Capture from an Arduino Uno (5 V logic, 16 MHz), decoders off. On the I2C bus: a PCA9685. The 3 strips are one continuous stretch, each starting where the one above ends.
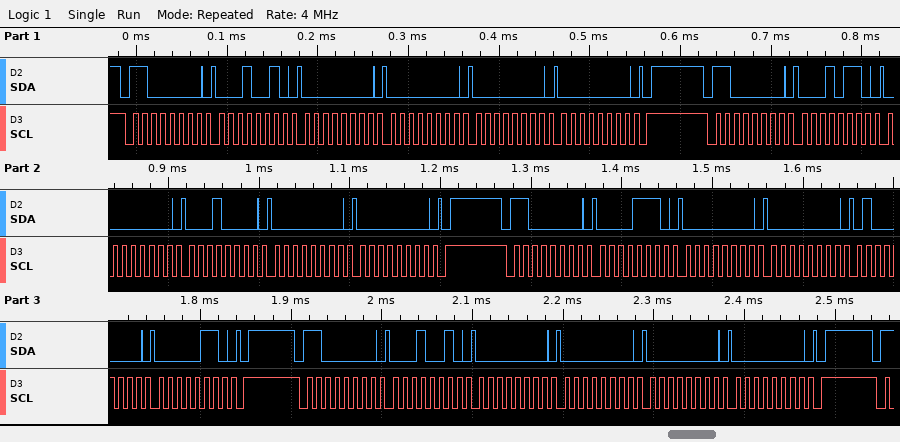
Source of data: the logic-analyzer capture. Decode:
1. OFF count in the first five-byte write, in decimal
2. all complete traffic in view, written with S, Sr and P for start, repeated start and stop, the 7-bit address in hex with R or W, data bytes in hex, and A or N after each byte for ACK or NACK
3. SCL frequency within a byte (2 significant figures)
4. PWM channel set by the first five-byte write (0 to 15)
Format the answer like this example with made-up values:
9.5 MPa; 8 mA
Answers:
0; S 60W A 12 A 00 A 00 A 00 A 00 A P S 60W A 16 A 00 A 10 A 00 A 00 A P S 60W A 0E A 00 A 00 A 40 A 06 A P S 60W A 12 A 00 A 00 A 00 A 00 A P; 100 kHz; 3
